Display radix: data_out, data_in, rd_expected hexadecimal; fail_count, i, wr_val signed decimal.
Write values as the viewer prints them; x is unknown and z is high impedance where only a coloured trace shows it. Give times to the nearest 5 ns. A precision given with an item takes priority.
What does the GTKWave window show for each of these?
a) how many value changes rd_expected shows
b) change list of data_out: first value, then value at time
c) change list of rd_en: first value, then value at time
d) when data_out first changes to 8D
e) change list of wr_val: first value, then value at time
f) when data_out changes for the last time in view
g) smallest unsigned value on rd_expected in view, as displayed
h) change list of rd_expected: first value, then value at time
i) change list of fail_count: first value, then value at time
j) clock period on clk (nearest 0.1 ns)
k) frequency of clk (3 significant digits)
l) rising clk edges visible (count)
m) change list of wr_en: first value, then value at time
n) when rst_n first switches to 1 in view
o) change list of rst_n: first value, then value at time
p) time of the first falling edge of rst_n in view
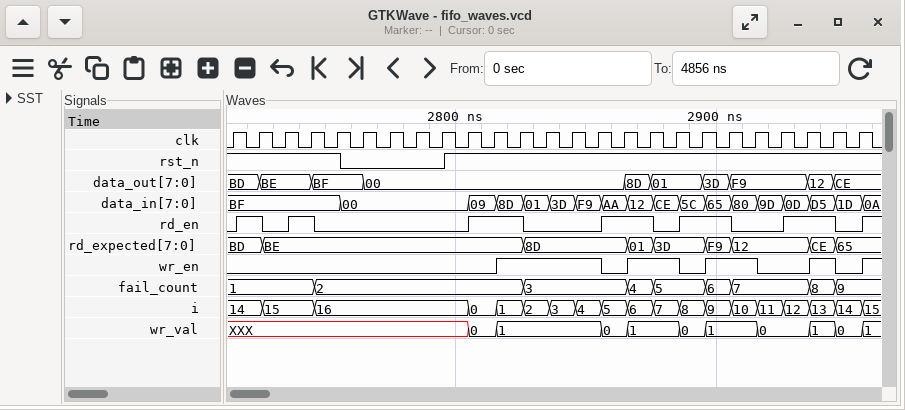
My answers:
8
BD, BE at 2725 ns, BF at 2745 ns, 00 at 2765 ns, 8D at 2865 ns, 01 at 2875 ns, 3D at 2895 ns, F9 at 2905 ns, 12 at 2935 ns, CE at 2945 ns
0, 1 at 2715 ns, 0 at 2725 ns, 1 at 2735 ns, 0 at 2745 ns, 1 at 2805 ns, 0 at 2825 ns, 1 at 2855 ns, 0 at 2875 ns, 1 at 2885 ns, 0 at 2905 ns, 1 at 2925 ns, 0 at 2945 ns, 1 at 2955 ns
2865 ns
XXX, 0 at 2805 ns, 1 at 2815 ns, 0 at 2855 ns, 1 at 2865 ns, 0 at 2885 ns, 1 at 2895 ns, 0 at 2915 ns, 1 at 2935 ns, 0 at 2945 ns, 1 at 2955 ns
2945 ns
01
BD, BE at 2725 ns, 8D at 2825 ns, 01 at 2865 ns, 3D at 2875 ns, F9 at 2895 ns, 12 at 2905 ns, CE at 2935 ns, 65 at 2945 ns
1, 2 at 2745 ns, 3 at 2825 ns, 4 at 2865 ns, 5 at 2875 ns, 6 at 2895 ns, 7 at 2905 ns, 8 at 2935 ns, 9 at 2945 ns
10 ns
100 MHz
25
0, 1 at 2815 ns, 0 at 2855 ns, 1 at 2865 ns, 0 at 2885 ns, 1 at 2895 ns, 0 at 2915 ns, 1 at 2935 ns, 0 at 2945 ns, 1 at 2955 ns
2795 ns
1, 0 at 2755 ns, 1 at 2795 ns
2755 ns
